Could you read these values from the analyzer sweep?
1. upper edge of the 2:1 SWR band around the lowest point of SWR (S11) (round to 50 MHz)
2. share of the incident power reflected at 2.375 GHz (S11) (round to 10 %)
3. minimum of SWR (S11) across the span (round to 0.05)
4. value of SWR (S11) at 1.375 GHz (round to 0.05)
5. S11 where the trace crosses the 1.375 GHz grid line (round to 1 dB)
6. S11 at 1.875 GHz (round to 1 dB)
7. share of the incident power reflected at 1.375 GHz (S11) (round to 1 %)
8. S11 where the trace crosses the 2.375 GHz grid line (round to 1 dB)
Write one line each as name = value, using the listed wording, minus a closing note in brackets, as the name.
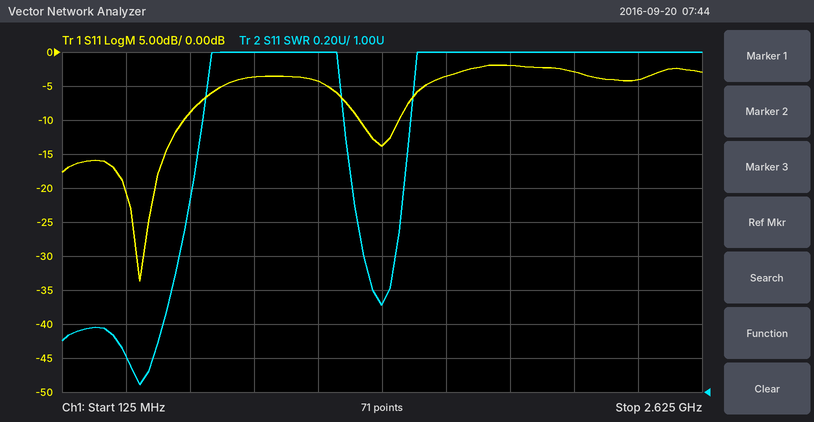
upper edge of the 2:1 SWR band around the lowest point of SWR (S11) = 600 MHz
share of the incident power reflected at 2.375 GHz (S11) = 40 %
minimum of SWR (S11) across the span = 1.05
value of SWR (S11) at 1.375 GHz = 1.50
S11 where the trace crosses the 1.375 GHz grid line = -14 dB
S11 at 1.875 GHz = -2 dB
share of the incident power reflected at 1.375 GHz (S11) = 4 %
S11 where the trace crosses the 2.375 GHz grid line = -4 dB
